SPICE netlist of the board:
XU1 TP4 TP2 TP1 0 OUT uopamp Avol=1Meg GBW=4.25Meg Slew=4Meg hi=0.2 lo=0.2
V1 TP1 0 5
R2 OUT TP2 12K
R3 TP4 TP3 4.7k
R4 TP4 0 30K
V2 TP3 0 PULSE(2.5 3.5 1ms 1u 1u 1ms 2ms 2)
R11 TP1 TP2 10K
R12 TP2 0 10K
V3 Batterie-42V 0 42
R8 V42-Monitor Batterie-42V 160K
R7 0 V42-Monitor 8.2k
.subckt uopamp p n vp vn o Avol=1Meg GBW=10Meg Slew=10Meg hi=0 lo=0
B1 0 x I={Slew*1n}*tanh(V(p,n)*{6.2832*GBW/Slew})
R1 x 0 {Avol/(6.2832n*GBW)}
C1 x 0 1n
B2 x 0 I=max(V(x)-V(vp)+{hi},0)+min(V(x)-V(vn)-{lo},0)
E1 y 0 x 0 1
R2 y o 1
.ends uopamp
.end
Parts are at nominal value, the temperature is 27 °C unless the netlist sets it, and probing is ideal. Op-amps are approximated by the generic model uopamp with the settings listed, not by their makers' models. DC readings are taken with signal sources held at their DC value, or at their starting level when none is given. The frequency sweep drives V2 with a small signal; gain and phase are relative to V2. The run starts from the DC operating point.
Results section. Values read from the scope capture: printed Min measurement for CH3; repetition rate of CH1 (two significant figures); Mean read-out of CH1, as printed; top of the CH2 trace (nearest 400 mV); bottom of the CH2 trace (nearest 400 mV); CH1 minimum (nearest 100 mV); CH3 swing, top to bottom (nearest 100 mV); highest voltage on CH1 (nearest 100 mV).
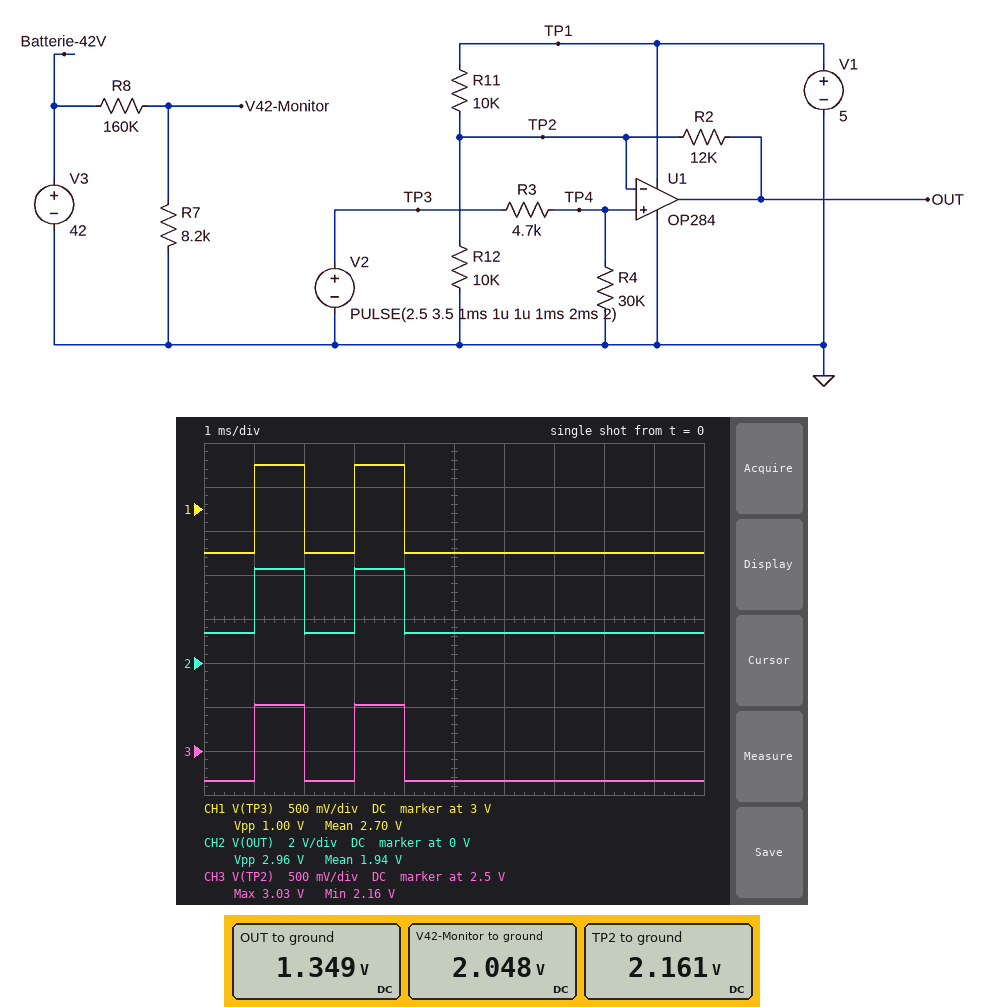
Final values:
2.16 V
500 Hz
2.70 V
4.4 V
1.2 V
2.5 V
900 mV
3.5 V
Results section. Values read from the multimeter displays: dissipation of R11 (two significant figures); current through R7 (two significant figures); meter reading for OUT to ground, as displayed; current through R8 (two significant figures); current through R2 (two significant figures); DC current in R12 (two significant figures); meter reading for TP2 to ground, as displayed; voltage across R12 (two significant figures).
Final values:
810 µW
250 µA
1.349 V
250 µA
68 µA
220 µA
2.161 V
2.2 V
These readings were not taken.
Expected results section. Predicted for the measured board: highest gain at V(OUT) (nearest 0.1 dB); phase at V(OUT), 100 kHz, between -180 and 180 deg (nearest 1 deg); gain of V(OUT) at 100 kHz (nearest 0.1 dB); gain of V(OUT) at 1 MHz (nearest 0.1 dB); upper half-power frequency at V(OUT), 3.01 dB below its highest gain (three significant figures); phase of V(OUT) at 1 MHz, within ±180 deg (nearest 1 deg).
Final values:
9.4 dB
-5 deg
9.3 dB
7.2 dB
1.25 MHz
-39 deg
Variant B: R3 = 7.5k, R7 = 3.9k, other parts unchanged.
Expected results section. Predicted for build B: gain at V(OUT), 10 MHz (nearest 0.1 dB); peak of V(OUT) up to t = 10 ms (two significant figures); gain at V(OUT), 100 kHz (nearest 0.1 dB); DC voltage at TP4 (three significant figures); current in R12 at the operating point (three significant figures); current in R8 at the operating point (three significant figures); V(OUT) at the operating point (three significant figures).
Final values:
-9.4 dB
3.5 V
8.7 dB
2.00 V
200 µA
256 µA
800 mV
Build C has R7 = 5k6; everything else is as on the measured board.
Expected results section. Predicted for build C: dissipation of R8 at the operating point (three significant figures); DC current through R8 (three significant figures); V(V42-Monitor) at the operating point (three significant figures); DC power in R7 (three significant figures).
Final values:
10.3 mW
254 µA
1.42 V
360 µW
